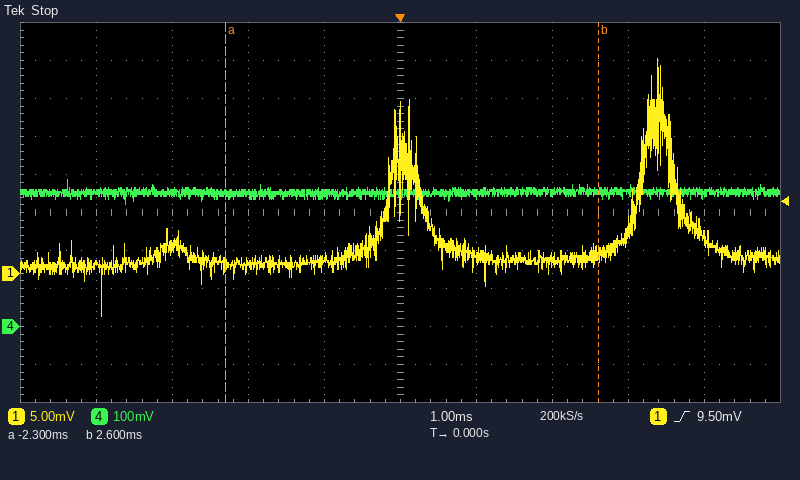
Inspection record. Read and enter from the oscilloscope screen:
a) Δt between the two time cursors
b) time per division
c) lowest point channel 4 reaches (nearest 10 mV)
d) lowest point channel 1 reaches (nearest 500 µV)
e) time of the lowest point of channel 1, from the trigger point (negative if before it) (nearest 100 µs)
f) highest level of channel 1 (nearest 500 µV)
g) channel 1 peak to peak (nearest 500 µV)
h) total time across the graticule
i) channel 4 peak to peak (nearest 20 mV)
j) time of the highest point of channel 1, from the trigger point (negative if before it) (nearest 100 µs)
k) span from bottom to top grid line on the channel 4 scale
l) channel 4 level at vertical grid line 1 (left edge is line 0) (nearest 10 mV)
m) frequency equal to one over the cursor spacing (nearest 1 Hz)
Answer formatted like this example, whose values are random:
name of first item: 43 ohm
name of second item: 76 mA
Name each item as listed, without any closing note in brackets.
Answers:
Δt between the two time cursors: 4.9 ms
time per division: 1 ms
lowest point channel 4 reaches: 320 mV
lowest point channel 1 reaches: -5.5 mV
time of the lowest point of channel 1, from the trigger point (negative if before it): -3.9 ms
highest level of channel 1: 28.5 mV
channel 1 peak to peak: 34.0 mV
total time across the graticule: 10 ms
channel 4 peak to peak: 60 mV
time of the highest point of channel 1, from the trigger point (negative if before it): +3.4 ms
span from bottom to top grid line on the channel 4 scale: 1 V
channel 4 level at vertical grid line 1 (left edge is line 0): 350 mV
frequency equal to one over the cursor spacing: 204 Hz
